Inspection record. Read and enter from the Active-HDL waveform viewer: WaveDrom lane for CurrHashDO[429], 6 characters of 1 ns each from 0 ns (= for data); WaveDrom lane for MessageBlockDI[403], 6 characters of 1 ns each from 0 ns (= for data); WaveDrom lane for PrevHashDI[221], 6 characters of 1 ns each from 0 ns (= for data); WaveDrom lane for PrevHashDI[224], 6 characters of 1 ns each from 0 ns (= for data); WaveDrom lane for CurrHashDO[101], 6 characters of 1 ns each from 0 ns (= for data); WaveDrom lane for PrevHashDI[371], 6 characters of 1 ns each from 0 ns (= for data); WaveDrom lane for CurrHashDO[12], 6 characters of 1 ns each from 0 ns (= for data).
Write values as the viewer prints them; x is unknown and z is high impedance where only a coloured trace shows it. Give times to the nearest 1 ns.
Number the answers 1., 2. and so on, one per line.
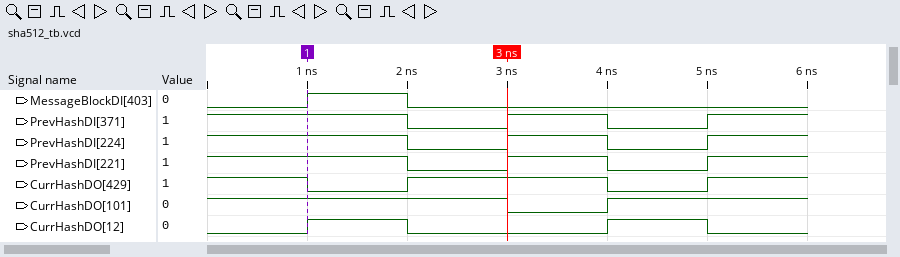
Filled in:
1. {name: 'CurrHashDO[429]', wave: '101.01'}
2. {name: 'MessageBlockDI[403]', wave: '010...'}
3. {name: 'PrevHashDI[221]', wave: '1.0101'}
4. {name: 'PrevHashDI[224]', wave: '1.0101'}
5. {name: 'CurrHashDO[101]', wave: '1..01.'}
6. {name: 'PrevHashDI[371]', wave: '1.0101'}
7. {name: 'CurrHashDO[12]', wave: '010.10'}
